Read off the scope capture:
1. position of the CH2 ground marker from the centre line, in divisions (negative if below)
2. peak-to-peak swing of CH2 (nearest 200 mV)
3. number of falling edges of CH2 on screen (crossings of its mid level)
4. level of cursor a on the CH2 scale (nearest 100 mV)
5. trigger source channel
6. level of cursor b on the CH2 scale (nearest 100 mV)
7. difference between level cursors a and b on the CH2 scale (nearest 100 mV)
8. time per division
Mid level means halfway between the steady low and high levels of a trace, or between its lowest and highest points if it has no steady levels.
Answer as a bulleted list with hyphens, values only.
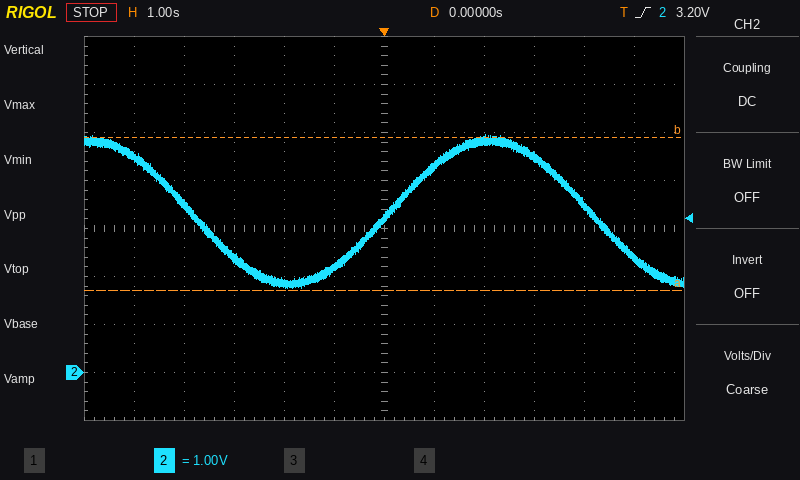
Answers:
- -3.0 div
- 3.2 V
- 2
- 1.7 V
- CH2
- 4.9 V
- 3.2 V
- 1 s
